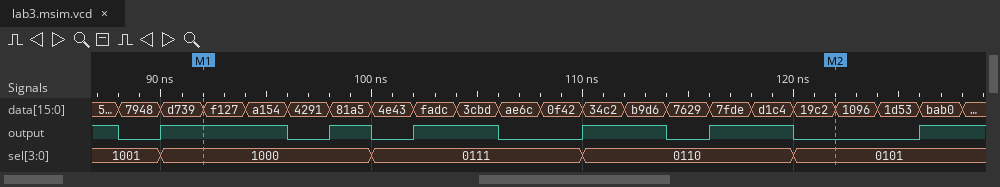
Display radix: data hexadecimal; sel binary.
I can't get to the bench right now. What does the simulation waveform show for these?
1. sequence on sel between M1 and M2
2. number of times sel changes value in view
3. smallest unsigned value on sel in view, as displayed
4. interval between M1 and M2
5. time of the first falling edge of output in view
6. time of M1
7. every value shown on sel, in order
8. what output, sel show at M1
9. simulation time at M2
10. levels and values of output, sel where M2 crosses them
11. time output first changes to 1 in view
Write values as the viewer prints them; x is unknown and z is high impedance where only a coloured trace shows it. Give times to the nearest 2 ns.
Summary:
1000, 0111, 0110, 0101
4
0101
30 ns
88 ns
92 ns
1001, 1000, 0111, 0110, 0101
output=1, sel=1000
122 ns
output=0, sel=0101
90 ns
